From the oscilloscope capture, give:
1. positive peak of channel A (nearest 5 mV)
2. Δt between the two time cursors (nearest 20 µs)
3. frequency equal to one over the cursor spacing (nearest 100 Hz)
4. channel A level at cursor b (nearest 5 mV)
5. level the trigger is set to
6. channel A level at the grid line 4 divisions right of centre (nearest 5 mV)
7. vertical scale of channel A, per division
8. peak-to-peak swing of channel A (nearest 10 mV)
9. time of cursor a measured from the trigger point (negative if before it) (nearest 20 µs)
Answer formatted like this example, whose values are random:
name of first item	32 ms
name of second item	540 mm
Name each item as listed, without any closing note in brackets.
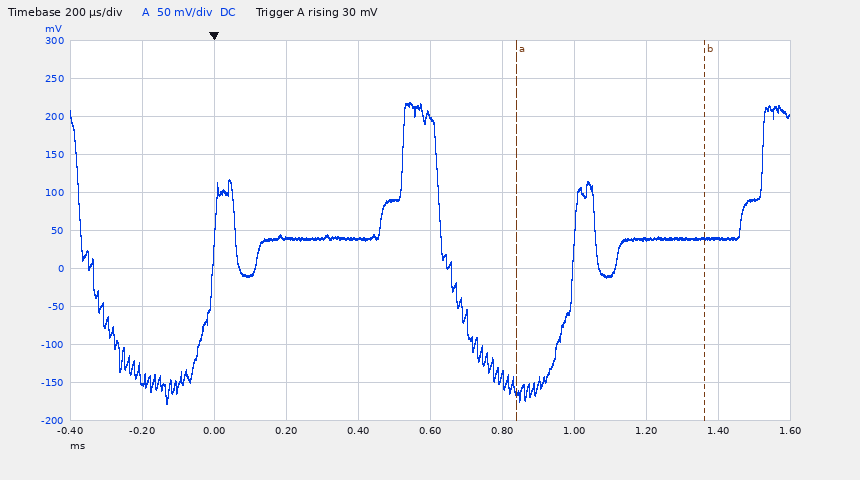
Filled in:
positive peak of channel A	220 mV
Δt between the two time cursors	520 µs
frequency equal to one over the cursor spacing	1.9 kHz
channel A level at cursor b	40 mV
level the trigger is set to	30 mV
channel A level at the grid line 4 divisions right of centre	40 mV
vertical scale of channel A, per division	50 mV
peak-to-peak swing of channel A	400 mV
time of cursor a measured from the trigger point (negative if before it)	+840 µs
